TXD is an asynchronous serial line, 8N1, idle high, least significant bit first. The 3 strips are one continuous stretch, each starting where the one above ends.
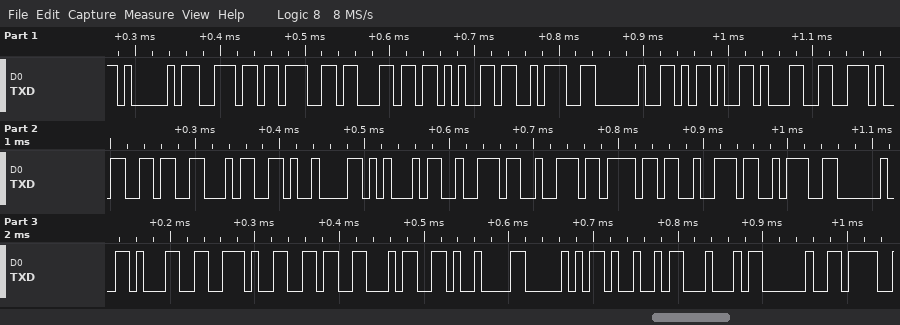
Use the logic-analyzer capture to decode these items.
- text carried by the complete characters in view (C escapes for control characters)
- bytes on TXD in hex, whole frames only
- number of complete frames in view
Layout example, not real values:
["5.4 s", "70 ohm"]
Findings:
["\"Angle: -1.64\\tError: 1.64\\tPID \"", "41 6E 67 6C 65 3A 20 2D 31 2E 36 34 09 45 72 72 6F 72 3A 20 31 2E 36 34 09 50 49 44 20", "29"]
